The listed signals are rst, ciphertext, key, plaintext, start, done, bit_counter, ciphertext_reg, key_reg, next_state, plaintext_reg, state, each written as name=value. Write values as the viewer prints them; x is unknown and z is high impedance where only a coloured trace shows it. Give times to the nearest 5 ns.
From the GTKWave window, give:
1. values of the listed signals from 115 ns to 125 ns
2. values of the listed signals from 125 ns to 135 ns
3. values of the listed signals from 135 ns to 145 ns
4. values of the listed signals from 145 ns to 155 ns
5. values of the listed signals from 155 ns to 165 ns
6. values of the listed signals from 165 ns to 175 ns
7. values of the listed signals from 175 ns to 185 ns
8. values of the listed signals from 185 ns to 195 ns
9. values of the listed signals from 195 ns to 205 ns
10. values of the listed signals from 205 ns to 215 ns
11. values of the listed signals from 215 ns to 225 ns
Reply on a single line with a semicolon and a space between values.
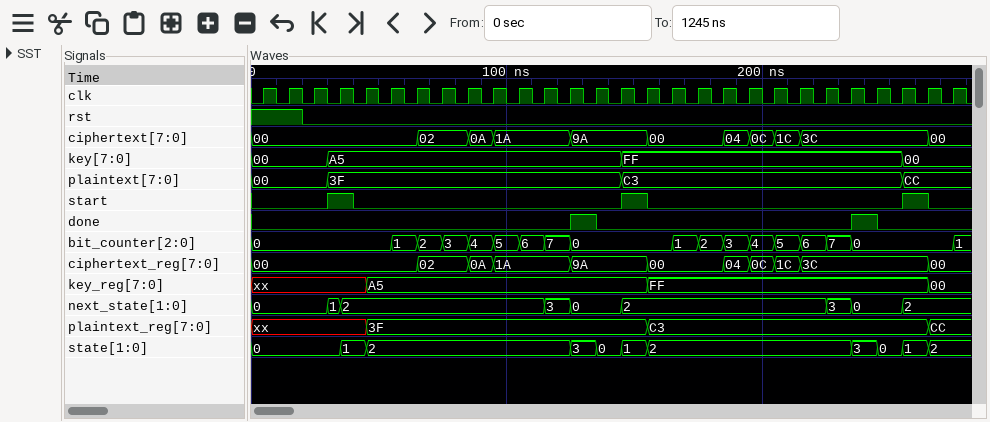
rst=0, ciphertext=1A, key=A5, plaintext=3F, start=0, done=0, bit_counter=7, ciphertext_reg=1A, key_reg=A5, next_state=3, plaintext_reg=3F, state=2; rst=0, ciphertext=9A, key=A5, plaintext=3F, start=0, done=1, bit_counter=0, ciphertext_reg=9A, key_reg=A5, next_state=0, plaintext_reg=3F, state=3; rst=0, ciphertext=9A, key=A5, plaintext=3F, start=0, done=0, bit_counter=0, ciphertext_reg=9A, key_reg=A5, next_state=0, plaintext_reg=3F, state=0; rst=0, ciphertext=9A, key=FF, plaintext=C3, start=1, done=0, bit_counter=0, ciphertext_reg=9A, key_reg=A5, next_state=2, plaintext_reg=3F, state=1; rst=0, ciphertext=00, key=FF, plaintext=C3, start=0, done=0, bit_counter=0, ciphertext_reg=00, key_reg=FF, next_state=2, plaintext_reg=C3, state=2; rst=0, ciphertext=00, key=FF, plaintext=C3, start=0, done=0, bit_counter=1, ciphertext_reg=00, key_reg=FF, next_state=2, plaintext_reg=C3, state=2; rst=0, ciphertext=00, key=FF, plaintext=C3, start=0, done=0, bit_counter=2, ciphertext_reg=00, key_reg=FF, next_state=2, plaintext_reg=C3, state=2; rst=0, ciphertext=04, key=FF, plaintext=C3, start=0, done=0, bit_counter=3, ciphertext_reg=04, key_reg=FF, next_state=2, plaintext_reg=C3, state=2; rst=0, ciphertext=0C, key=FF, plaintext=C3, start=0, done=0, bit_counter=4, ciphertext_reg=0C, key_reg=FF, next_state=2, plaintext_reg=C3, state=2; rst=0, ciphertext=1C, key=FF, plaintext=C3, start=0, done=0, bit_counter=5, ciphertext_reg=1C, key_reg=FF, next_state=2, plaintext_reg=C3, state=2; rst=0, ciphertext=3C, key=FF, plaintext=C3, start=0, done=0, bit_counter=6, ciphertext_reg=3C, key_reg=FF, next_state=2, plaintext_reg=C3, state=2
